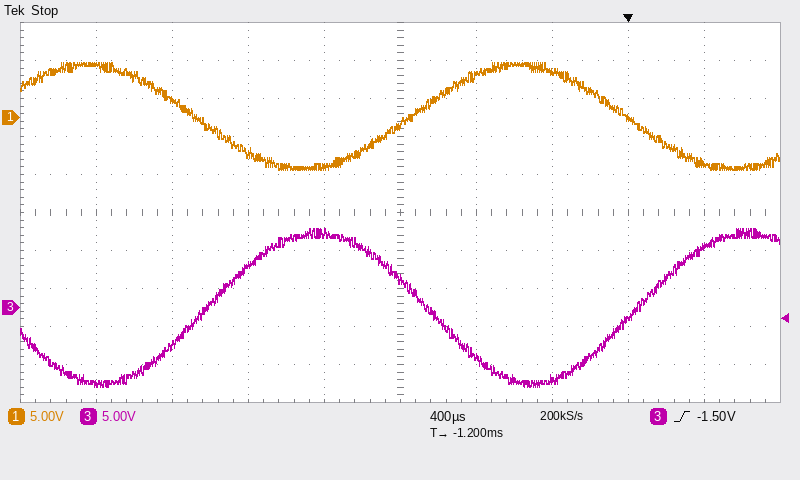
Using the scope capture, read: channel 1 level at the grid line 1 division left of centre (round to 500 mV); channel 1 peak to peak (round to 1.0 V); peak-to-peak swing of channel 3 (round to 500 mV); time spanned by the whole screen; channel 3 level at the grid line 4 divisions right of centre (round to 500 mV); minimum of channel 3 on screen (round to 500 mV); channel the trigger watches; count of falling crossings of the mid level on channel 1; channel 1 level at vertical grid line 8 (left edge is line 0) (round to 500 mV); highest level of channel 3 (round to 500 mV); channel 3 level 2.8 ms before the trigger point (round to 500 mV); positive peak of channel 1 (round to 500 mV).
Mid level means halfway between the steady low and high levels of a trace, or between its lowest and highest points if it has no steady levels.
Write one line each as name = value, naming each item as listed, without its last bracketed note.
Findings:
channel 1 level at the grid line 1 division left of centre = -6.5 V
channel 1 peak to peak = 14.0 V
peak-to-peak swing of channel 3 = 21.0 V
time spanned by the whole screen = 4 ms
channel 3 level at the grid line 4 divisions right of centre = 8.0 V
minimum of channel 3 on screen = -10.5 V
channel the trigger watches = channel 3
count of falling crossings of the mid level on channel 1 = 2
channel 1 level at vertical grid line 8 (left edge is line 0) = 0.0 V
highest level of channel 3 = 10.5 V
channel 3 level 2.8 ms before the trigger point = -10.0 V
positive peak of channel 1 = 7.0 V
